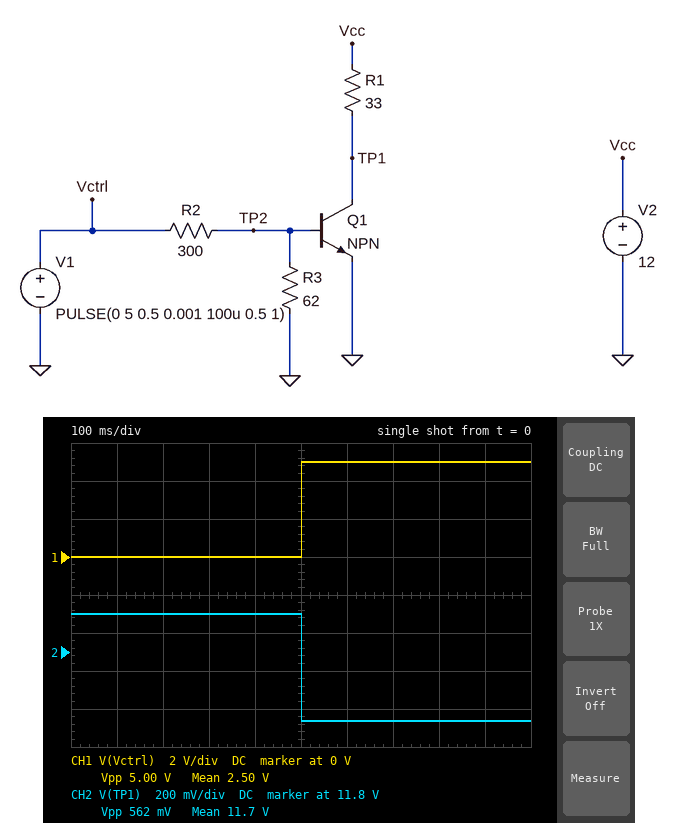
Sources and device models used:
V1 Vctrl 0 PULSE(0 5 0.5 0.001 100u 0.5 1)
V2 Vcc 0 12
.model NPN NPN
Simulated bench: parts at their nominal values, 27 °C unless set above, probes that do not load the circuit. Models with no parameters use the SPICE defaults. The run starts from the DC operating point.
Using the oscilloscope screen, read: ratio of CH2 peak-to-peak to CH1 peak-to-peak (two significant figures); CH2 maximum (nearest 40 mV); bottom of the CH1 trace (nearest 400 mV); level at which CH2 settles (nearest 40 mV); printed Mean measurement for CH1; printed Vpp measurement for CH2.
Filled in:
0.11
12.00 V
0 V
11.44 V
2.50 V
562 mV
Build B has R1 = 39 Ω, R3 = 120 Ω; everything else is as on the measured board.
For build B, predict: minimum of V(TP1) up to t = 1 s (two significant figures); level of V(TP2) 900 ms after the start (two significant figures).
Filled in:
120 mV
920 mV
